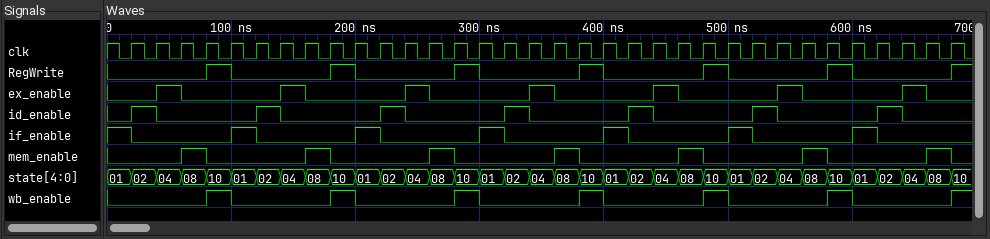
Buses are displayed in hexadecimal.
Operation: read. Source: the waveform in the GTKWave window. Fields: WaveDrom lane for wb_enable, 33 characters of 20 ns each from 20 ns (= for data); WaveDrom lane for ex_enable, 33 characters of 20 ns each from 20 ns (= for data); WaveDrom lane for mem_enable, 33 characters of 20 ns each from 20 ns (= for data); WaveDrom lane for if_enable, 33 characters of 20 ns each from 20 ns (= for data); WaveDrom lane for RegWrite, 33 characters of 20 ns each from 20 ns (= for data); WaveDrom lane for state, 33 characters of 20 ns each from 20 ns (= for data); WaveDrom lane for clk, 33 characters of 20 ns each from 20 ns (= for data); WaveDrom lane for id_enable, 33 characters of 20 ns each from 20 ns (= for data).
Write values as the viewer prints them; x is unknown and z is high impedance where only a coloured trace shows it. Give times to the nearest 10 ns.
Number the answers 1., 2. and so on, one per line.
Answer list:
1. {name: 'wb_enable', wave: '0..10...10...10...10...10...10...'}
2. {name: 'ex_enable', wave: '010...10...10...10...10...10...10'}
3. {name: 'mem_enable', wave: '0.10...10...10...10...10...10...1'}
4. {name: 'if_enable', wave: '0...10...10...10...10...10...10..'}
5. {name: 'RegWrite', wave: '0..10...10...10...10...10...10...'}
6. {name: 'state', wave: '=================================', data: '02 04 08 10 01 02 04 08 10 01 02 04 08 10 01 02 04 08 10 01 02 04 08 10 01 02 04 08 10 01 02 04 08'}
7. {name: 'clk', wave: 'p................................'}
8. {name: 'id_enable', wave: '10...10...10...10...10...10...10.'}
